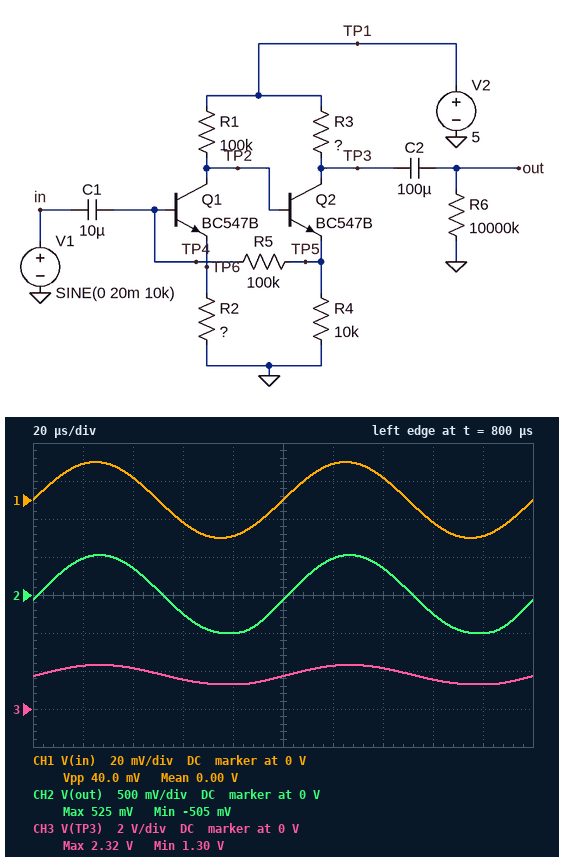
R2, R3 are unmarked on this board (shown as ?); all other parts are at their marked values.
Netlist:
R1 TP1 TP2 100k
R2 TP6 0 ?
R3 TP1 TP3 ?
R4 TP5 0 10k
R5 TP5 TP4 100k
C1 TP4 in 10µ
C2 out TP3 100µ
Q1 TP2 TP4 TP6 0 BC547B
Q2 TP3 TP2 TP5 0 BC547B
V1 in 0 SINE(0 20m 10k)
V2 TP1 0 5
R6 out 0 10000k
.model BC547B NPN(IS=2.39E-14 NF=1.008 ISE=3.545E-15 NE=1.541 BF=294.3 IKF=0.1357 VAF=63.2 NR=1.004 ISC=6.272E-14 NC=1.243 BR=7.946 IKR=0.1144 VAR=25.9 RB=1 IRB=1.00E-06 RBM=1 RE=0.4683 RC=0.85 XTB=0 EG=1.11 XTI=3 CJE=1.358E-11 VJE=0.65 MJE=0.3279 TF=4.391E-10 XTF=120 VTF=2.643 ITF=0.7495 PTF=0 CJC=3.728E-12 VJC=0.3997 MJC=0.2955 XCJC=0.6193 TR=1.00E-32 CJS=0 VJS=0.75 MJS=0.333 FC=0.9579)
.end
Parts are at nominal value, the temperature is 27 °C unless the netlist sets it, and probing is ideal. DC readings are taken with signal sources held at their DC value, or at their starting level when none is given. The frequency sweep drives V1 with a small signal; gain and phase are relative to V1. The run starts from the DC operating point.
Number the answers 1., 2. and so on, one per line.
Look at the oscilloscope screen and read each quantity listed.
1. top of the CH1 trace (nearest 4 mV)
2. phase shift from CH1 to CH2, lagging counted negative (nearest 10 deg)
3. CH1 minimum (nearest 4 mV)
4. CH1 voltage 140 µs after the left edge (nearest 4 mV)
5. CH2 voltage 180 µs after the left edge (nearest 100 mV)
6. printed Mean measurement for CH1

1. 20 mV
2. -10 deg
3. -20 mV
4. 12 mV
5. -500 mV
6. 0.00 V
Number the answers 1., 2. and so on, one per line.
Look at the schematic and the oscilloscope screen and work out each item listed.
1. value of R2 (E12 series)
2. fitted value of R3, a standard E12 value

1. 12 kΩ
2. 33 kΩ
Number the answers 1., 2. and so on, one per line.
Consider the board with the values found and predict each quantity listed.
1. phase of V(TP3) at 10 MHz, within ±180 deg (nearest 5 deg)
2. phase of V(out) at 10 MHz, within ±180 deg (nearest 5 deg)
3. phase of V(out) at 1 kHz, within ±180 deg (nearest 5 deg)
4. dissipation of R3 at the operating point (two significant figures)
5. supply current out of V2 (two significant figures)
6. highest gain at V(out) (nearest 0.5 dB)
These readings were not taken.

1. 70 deg
2. 70 deg
3. 0 deg
4. 310 µW
5. 130 µA
6. 28.5 dB
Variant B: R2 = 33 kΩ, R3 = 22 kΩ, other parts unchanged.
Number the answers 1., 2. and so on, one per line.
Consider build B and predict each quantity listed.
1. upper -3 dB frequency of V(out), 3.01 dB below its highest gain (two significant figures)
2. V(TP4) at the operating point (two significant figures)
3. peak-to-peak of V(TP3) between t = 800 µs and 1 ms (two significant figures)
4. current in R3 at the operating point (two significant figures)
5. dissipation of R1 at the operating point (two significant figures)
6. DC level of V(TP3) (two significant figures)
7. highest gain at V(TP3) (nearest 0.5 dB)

1. 54 kHz
2. 1.5 V
3. 190 mV
4. 150 µA
5. 85 µW
6. 1.7 V
7. 15.0 dB
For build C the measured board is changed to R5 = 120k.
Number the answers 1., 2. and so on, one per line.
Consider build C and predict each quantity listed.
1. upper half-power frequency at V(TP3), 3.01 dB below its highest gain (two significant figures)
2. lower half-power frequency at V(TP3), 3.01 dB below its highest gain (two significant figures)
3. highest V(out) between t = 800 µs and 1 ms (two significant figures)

1. 87 kHz
2. 1.1 Hz
3. 520 mV
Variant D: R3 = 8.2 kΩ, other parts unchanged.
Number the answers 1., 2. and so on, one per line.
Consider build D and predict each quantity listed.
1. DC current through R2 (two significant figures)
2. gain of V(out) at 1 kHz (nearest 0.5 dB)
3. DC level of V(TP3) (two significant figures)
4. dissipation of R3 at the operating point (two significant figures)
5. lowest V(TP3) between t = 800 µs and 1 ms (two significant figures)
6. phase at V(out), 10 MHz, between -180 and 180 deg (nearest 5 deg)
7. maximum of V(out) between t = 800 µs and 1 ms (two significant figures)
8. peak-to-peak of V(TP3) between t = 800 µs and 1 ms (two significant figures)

1. 34 µA
2. 16.5 dB
3. 4.2 V
4. 77 µW
5. 4.1 V
6. 105 deg
7. 130 mV
8. 260 mV
